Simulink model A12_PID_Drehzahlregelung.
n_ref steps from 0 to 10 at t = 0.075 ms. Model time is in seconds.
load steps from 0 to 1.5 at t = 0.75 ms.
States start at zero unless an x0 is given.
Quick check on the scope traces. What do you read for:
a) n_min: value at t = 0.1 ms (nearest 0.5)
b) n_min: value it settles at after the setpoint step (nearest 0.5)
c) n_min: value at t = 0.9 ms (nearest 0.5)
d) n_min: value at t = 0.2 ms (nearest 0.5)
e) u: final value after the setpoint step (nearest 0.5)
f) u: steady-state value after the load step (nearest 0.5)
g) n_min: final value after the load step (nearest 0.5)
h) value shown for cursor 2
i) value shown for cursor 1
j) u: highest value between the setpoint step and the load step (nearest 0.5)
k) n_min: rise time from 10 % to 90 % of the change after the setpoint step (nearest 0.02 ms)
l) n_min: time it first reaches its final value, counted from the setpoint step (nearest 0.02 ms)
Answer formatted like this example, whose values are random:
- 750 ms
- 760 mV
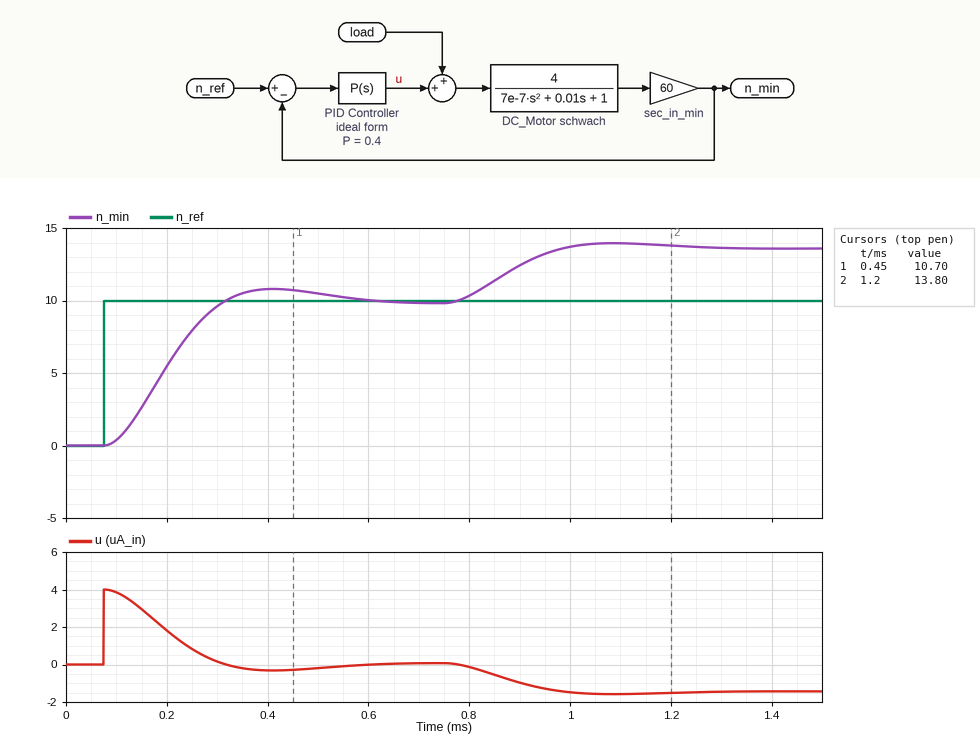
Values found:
- 0.5
- 10.0
- 12.5
- 5.5
- 0.0
- -1.5
- 13.5
- 13.80
- 10.70
- 4.0
- 0.16 ms
- 0.24 ms
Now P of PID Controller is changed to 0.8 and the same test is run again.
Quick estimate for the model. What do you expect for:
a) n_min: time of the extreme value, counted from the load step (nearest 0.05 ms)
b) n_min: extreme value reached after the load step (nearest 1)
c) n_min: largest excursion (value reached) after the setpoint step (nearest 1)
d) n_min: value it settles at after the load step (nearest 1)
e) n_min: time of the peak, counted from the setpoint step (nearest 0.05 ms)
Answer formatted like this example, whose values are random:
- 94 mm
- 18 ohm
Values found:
- 0.20 ms
- 12
- 12
- 12
- 0.20 ms
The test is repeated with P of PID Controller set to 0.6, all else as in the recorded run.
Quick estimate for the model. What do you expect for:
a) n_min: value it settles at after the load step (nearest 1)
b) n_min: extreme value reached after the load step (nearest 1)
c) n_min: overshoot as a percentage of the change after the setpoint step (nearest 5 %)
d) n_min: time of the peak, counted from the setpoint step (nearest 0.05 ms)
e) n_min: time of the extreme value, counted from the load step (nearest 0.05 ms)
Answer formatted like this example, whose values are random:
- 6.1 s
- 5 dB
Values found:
- 12
- 13
- 15 %
- 0.25 ms
- 0.25 ms
